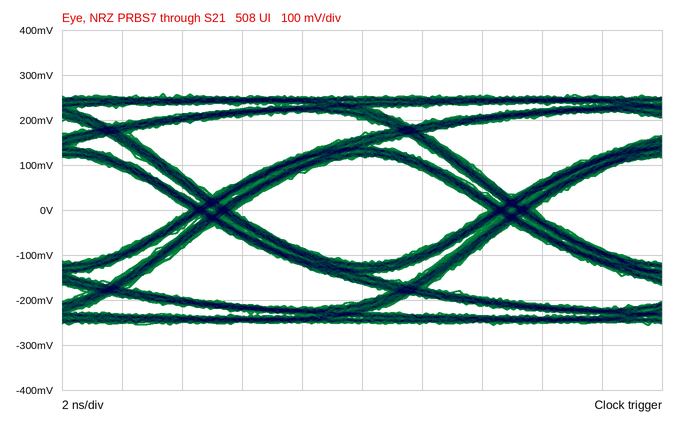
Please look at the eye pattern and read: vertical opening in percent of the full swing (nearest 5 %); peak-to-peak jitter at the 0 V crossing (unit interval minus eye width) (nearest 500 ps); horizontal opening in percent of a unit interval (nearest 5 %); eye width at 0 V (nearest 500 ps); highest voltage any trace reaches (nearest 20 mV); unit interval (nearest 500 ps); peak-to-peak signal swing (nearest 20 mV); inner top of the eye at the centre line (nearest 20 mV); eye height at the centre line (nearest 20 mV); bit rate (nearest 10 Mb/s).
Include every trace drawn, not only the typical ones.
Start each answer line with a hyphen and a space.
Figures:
- 45 %
- 1.5 ns
- 85 %
- 8.5 ns
- 260 mV
- 10.0 ns
- 520 mV
- 120 mV
- 240 mV
- 100 Mb/s
